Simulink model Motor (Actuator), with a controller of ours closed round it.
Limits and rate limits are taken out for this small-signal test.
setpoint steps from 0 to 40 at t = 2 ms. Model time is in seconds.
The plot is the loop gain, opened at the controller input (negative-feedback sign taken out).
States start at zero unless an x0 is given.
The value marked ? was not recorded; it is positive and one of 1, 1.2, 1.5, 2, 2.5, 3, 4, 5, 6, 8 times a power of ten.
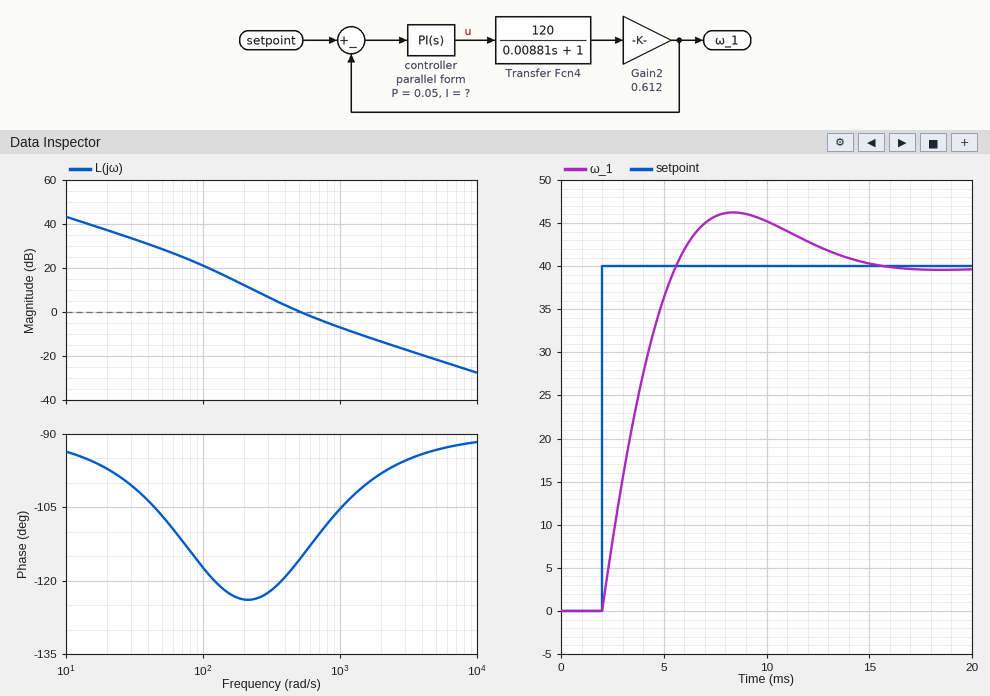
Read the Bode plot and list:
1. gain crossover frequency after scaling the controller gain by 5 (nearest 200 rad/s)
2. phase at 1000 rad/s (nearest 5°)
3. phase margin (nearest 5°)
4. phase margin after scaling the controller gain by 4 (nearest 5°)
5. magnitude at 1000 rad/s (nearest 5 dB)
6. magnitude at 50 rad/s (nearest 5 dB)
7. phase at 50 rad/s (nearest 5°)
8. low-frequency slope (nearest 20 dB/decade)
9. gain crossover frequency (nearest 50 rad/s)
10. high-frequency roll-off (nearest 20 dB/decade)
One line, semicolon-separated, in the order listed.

2200 rad/s; -105°; 65°; 80°; -5 dB; 30 dB; -105°; -20 dB/decade; 500 rad/s; -20 dB/decade
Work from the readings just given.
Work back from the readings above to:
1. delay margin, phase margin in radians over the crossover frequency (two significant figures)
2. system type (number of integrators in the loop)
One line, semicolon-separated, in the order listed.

0.0023 s; 1
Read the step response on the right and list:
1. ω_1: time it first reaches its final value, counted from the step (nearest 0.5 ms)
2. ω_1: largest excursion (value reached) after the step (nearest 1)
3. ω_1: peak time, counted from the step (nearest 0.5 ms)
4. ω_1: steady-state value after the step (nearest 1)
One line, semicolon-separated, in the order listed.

3.5 ms; 46; 6.5 ms; 40
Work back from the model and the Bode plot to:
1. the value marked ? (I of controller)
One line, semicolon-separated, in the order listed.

20
